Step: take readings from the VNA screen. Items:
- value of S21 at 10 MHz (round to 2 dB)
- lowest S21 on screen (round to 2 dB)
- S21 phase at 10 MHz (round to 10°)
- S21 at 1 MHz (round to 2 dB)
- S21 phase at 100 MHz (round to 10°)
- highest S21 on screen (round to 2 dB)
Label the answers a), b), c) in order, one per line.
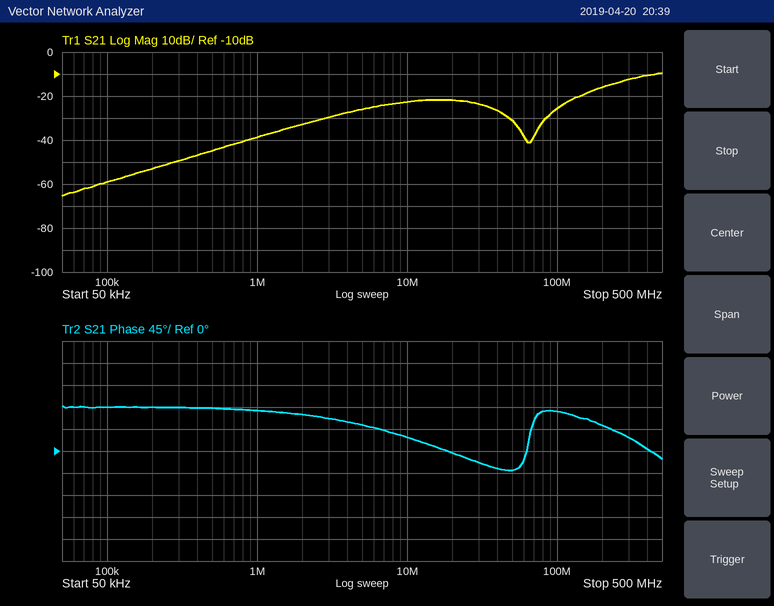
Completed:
a) -22 dB
b) -66 dB
c) 30°
d) -38 dB
e) 80°
f) -10 dB
